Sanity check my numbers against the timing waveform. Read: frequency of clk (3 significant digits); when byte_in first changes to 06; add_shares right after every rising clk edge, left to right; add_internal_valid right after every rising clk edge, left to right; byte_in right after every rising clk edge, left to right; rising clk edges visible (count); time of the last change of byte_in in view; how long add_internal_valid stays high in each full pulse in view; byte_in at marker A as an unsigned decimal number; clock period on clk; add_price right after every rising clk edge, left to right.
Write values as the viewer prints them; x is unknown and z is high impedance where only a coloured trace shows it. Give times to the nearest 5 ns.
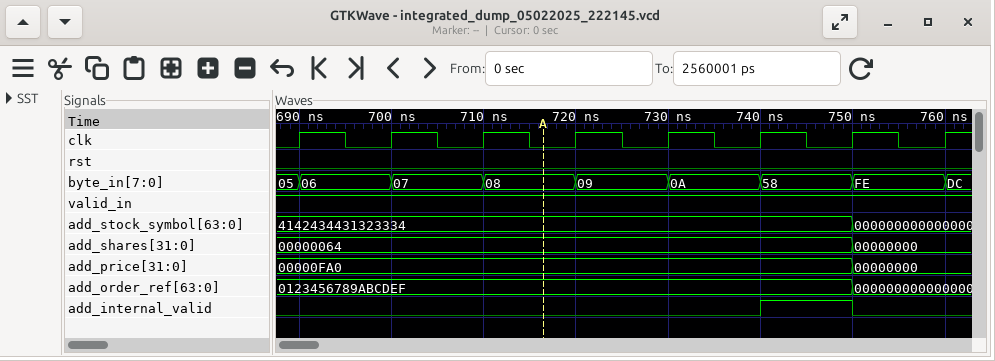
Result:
100 MHz
690 ns
00000064, 00000064, 00000064, 00000064, 00000064, 00000064, 00000000, 00000000
0 0 0 0 0 1 0 0
06, 07, 08, 09, 0A, 58, FE, DC
8
760 ns
10 ns
8
10 ns
00000FA0, 00000FA0, 00000FA0, 00000FA0, 00000FA0, 00000FA0, 00000000, 00000000
